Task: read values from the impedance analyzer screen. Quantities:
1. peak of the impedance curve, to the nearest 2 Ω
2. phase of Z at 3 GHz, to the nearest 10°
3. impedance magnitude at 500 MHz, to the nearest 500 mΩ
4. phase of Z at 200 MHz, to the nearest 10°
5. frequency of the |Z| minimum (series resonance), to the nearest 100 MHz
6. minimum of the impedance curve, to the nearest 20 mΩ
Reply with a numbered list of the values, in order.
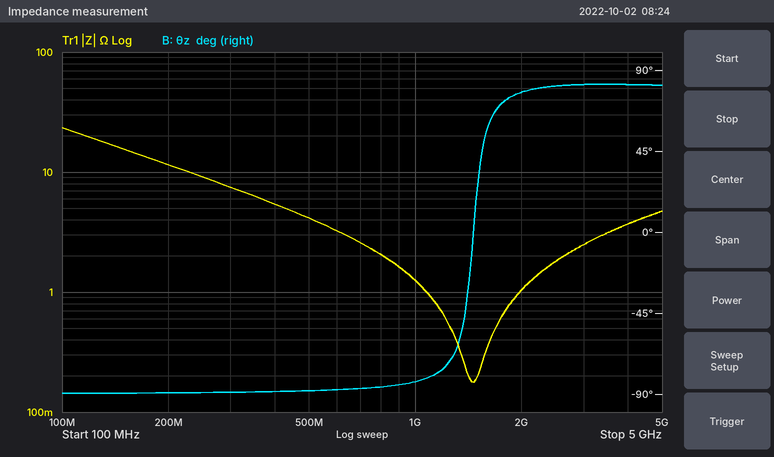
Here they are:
1. 24 Ω
2. 80°
3. 4.0 Ω
4. -90°
5. 1.5 GHz
6. 180 mΩ
